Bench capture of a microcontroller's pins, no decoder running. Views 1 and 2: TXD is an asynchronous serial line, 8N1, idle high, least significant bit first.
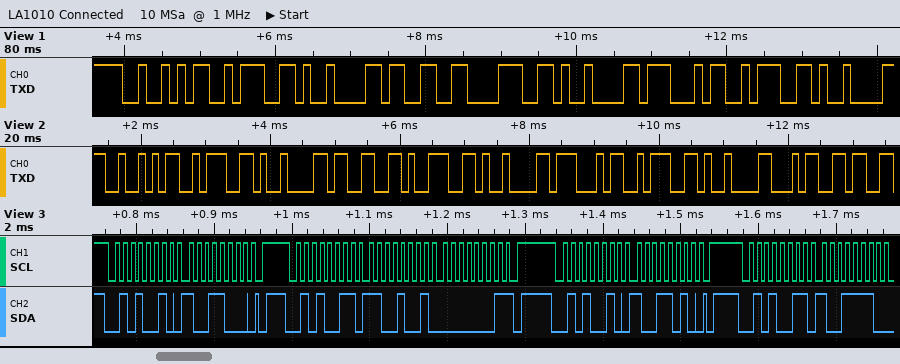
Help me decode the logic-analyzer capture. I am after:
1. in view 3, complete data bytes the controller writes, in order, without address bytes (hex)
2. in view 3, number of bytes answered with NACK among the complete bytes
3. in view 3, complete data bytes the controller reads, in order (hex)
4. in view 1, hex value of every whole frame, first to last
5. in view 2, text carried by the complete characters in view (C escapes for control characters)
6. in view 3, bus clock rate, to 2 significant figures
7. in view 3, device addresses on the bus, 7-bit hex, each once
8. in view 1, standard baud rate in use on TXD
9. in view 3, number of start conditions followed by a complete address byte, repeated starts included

98 9A
1
C9 01 9E
52 3A 09 33 38 09 47 3A 09
"R:\t39\tG:\t4"
100 kHz
0x29
9600 baud
4
